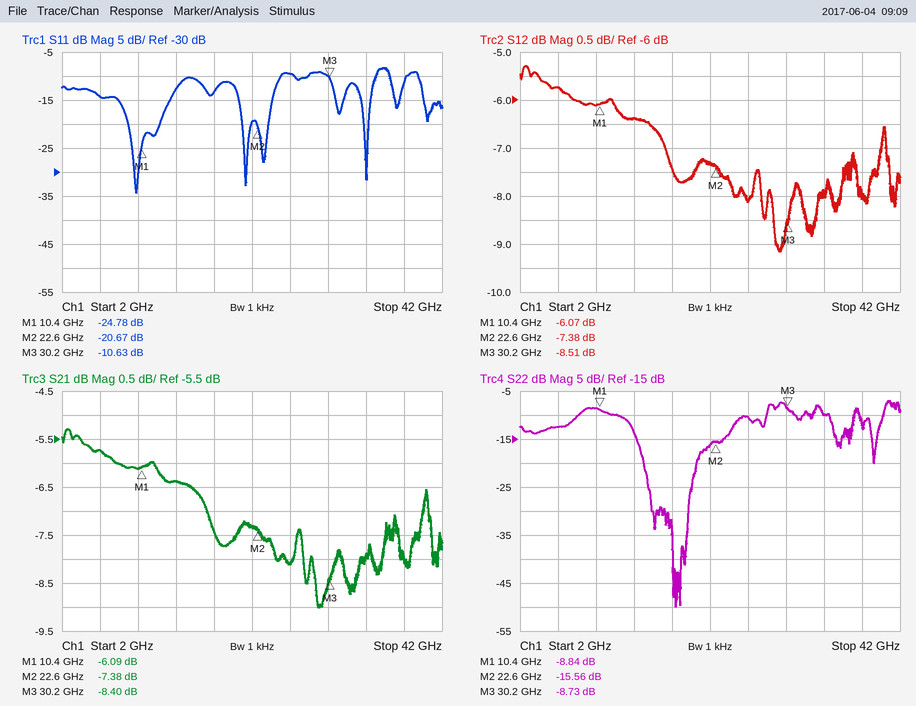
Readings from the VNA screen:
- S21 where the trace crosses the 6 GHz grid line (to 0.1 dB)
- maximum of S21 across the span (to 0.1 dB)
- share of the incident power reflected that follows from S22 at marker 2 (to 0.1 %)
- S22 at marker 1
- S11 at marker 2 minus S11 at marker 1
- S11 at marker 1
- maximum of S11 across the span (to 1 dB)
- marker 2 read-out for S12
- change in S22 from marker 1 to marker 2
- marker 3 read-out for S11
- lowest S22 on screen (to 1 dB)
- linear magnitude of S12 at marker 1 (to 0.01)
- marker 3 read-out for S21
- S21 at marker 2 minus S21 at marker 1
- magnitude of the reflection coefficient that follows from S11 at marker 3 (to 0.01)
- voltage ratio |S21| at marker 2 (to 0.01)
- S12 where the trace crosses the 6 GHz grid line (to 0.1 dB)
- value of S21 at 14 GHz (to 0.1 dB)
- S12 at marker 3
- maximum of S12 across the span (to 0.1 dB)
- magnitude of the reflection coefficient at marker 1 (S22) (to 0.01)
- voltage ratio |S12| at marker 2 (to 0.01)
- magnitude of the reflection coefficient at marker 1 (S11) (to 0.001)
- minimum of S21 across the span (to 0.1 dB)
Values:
-5.7 dB
-5.3 dB
2.8 %
-8.84 dB
4.11 dB
-24.78 dB
-8 dB
-7.38 dB
-6.72 dB
-10.63 dB
-50 dB
0.50
-8.40 dB
-1.29 dB
0.29
0.43
-5.7 dB
-6.4 dB
-8.51 dB
-5.3 dB
0.36
0.43
0.058
-9.0 dB
